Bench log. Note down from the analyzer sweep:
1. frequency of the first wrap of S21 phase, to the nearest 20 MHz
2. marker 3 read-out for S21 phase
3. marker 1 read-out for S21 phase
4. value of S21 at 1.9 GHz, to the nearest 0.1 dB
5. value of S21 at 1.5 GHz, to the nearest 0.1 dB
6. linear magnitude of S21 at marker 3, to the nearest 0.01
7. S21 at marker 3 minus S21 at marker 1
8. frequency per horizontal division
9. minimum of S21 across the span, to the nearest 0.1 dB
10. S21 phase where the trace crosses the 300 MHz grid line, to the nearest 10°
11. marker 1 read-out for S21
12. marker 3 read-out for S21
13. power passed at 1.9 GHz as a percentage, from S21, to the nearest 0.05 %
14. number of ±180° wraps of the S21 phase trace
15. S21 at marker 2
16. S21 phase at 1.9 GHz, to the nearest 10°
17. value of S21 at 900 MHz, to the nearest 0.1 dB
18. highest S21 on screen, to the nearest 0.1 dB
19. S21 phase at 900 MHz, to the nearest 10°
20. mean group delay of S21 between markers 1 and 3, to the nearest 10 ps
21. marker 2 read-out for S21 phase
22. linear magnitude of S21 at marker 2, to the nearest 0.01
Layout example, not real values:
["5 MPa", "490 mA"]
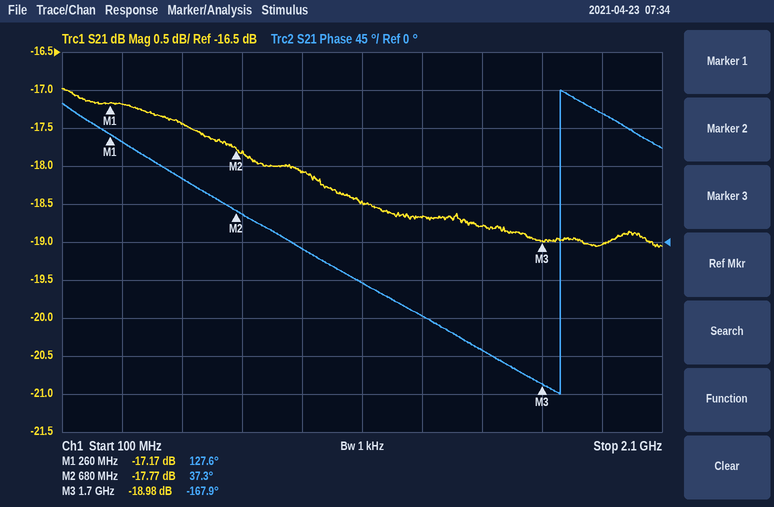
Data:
["1.76 GHz", "-167.9°", "127.6°", "-19.0 dB", "-18.8 dB", "0.11", "-1.81 dB", "200 MHz", "-19.1 dB", "120°", "-17.17 dB", "-18.98 dB", "1.25 %", "1", "-17.77 dB", "150°", "-18.1 dB", "-17.0 dB", "-10°", "570 ps", "37.3°", "0.13"]
